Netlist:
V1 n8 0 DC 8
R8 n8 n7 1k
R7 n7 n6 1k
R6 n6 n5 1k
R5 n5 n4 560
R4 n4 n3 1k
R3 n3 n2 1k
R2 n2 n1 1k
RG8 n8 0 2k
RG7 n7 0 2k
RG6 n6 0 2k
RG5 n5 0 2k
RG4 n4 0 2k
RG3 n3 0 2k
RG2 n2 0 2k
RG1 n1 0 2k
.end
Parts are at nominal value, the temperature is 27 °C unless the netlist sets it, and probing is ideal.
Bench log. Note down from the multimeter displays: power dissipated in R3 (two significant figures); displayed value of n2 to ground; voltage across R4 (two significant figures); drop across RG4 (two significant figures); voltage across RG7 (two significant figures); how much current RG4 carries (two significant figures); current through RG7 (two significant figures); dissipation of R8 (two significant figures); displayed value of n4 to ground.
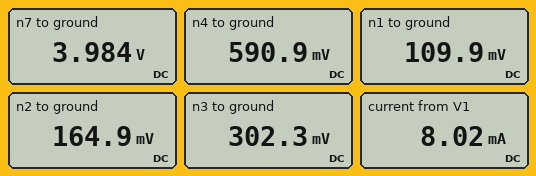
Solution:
19 µW
164.9 mV
290 mV
590 mV
4.0 V
300 µA
2.0 mA
16 mW
590.9 mV
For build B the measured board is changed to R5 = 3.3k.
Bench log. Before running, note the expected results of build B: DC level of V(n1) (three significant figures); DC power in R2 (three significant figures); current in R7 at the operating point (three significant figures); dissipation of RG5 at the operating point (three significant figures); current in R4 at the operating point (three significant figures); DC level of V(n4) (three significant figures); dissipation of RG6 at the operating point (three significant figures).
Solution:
53.0 mV
702 nW
1.94 mA
736 µW
139 µA
285 mV
2.21 mW
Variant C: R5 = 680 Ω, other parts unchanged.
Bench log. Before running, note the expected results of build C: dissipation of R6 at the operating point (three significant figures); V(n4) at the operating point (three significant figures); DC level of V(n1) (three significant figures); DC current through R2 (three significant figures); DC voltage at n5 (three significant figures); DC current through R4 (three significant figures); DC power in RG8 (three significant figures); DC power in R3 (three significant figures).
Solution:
1.06 mW
564 mV
105 mV
52.5 µA
944 mV
276 µA
32.0 mW
17.2 µW
